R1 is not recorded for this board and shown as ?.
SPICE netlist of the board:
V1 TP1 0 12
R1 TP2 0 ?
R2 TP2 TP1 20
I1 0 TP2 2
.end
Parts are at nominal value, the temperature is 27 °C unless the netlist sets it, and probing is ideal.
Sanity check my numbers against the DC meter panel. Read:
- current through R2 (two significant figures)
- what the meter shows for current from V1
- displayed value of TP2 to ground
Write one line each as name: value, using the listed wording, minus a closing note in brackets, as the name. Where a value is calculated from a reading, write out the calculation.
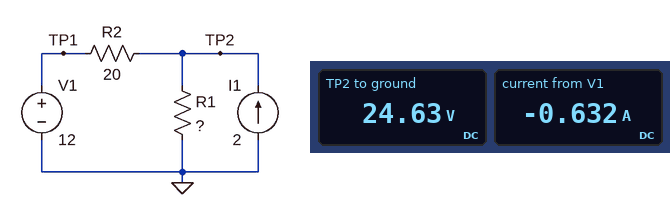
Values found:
current through R2: (24.63 V - 12 V) / 20 Ω = 630 mA
what the meter shows for current from V1: -0.632 A
displayed value of TP2 to ground: 24.63 V
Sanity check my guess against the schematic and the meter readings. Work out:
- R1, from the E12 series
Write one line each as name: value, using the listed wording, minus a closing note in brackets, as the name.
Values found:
R1, from the E12 series: 18 Ω
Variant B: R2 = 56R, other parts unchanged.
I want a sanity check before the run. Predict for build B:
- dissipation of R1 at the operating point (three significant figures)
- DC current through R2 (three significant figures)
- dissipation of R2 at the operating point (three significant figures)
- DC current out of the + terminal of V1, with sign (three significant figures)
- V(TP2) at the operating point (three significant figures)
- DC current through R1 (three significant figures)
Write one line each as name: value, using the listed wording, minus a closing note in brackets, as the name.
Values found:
dissipation of R1 at the operating point: 50.5 W
DC current through R2: 324 mA
dissipation of R2 at the operating point: 5.89 W
DC current out of the + terminal of V1, with sign: -324 mA
V(TP2) at the operating point: 30.2 V
DC current through R1: 1.68 A
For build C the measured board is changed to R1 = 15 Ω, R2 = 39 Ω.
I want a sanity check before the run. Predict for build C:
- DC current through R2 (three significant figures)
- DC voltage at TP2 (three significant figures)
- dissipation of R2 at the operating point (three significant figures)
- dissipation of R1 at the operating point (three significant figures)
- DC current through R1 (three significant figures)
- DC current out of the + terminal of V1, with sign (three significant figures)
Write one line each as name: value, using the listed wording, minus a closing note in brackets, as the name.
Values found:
DC current through R2: 333 mA
DC voltage at TP2: 25.0 V
dissipation of R2 at the operating point: 4.33 W
dissipation of R1 at the operating point: 41.7 W
DC current through R1: 1.67 A
DC current out of the + terminal of V1, with sign: -333 mA
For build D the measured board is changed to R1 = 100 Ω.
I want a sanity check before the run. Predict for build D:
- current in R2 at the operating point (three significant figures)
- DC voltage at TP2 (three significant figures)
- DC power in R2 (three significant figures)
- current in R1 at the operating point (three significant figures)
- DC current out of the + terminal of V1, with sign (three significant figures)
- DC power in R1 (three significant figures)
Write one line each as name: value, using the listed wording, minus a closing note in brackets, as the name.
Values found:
current in R2 at the operating point: 1.57 A
DC voltage at TP2: 43.3 V
DC power in R2: 49.1 W
current in R1 at the operating point: 433 mA
DC current out of the + terminal of V1, with sign: -1.57 A
DC power in R1: 18.8 W
